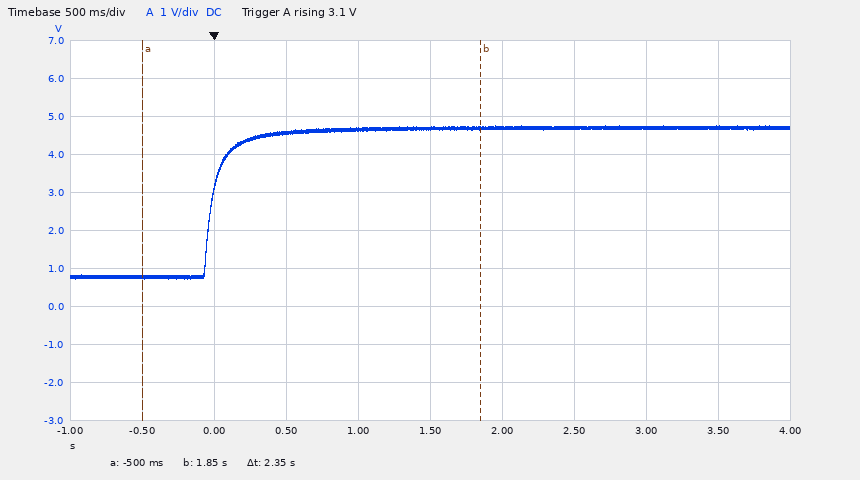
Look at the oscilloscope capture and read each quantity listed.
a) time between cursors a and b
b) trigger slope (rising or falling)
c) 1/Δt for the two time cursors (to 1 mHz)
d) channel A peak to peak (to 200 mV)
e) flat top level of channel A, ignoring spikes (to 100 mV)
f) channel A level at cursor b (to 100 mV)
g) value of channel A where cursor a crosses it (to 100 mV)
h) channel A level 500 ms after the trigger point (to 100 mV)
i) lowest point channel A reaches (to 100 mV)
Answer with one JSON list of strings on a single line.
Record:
["2.35 s", "rising", "426 mHz", "4.0 V", "4.7 V", "4.7 V", "800 mV", "4.6 V", "700 mV"]
